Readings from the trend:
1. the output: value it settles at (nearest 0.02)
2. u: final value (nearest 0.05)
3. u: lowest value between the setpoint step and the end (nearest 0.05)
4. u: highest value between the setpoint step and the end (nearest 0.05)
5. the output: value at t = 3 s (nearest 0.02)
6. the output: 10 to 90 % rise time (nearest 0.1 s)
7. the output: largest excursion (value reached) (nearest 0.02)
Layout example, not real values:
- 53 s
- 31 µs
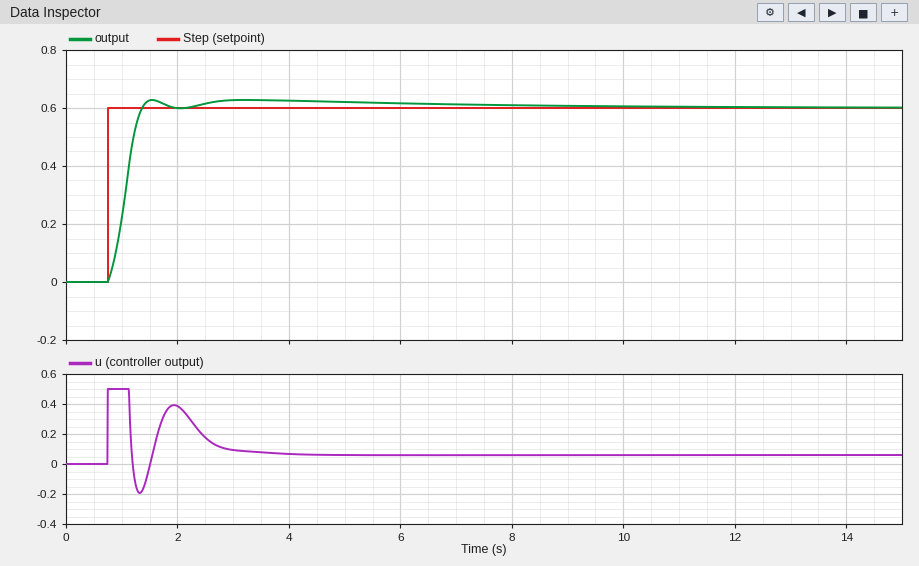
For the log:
- 0.60
- 0.05
- -0.20
- 0.50
- 0.62
- 0.4 s
- 0.62
